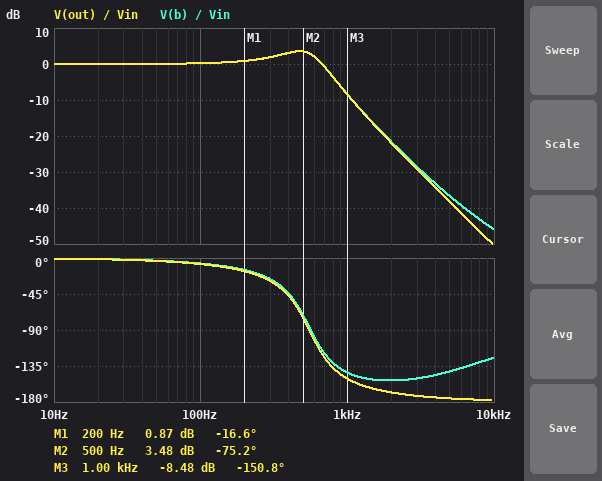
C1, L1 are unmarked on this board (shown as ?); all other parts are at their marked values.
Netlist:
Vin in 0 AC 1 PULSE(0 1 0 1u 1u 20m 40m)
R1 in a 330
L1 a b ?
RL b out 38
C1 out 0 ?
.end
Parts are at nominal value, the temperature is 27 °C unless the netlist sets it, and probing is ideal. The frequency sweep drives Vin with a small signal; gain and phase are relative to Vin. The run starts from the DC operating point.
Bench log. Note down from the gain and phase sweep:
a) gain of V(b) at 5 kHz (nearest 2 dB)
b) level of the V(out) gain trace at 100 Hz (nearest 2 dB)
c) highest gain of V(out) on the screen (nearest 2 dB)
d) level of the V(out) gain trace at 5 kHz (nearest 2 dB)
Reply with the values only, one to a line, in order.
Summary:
-36 dB
0 dB
4 dB
-38 dB
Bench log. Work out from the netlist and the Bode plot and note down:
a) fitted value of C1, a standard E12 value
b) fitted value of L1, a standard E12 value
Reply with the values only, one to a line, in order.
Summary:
560 nF
150 mH
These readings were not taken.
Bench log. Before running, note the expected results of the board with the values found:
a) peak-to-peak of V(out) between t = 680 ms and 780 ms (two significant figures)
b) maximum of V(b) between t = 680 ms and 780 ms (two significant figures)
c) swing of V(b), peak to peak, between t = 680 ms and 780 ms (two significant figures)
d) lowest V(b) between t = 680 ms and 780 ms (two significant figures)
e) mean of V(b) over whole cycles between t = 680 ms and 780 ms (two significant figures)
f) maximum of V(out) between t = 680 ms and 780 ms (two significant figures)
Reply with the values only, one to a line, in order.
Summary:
1.6 V
1.3 V
1.6 V
-310 mV
500 mV
1.3 V
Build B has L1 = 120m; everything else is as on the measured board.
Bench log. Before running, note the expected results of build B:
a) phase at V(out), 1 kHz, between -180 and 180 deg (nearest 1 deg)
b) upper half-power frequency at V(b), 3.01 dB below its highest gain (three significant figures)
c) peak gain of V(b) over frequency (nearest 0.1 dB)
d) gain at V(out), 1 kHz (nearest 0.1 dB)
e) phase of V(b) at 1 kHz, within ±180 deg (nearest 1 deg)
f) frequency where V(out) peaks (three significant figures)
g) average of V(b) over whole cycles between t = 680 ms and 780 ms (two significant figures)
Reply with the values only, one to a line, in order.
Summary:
-142 deg
731 Hz
2.8 dB
-6.4 dB
-134 deg
508 Hz
500 mV
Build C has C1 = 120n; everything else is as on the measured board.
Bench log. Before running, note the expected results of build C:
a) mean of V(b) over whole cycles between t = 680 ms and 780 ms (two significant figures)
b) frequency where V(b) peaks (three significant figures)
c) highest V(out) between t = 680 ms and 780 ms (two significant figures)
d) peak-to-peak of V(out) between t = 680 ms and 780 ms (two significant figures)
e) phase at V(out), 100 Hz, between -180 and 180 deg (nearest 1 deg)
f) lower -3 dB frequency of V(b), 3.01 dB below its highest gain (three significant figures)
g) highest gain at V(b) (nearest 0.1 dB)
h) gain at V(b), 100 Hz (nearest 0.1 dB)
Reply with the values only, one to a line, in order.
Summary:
500 mV
1.15 kHz
1.6 V
2.2 V
-2 deg
935 Hz
9.8 dB
0.1 dB
